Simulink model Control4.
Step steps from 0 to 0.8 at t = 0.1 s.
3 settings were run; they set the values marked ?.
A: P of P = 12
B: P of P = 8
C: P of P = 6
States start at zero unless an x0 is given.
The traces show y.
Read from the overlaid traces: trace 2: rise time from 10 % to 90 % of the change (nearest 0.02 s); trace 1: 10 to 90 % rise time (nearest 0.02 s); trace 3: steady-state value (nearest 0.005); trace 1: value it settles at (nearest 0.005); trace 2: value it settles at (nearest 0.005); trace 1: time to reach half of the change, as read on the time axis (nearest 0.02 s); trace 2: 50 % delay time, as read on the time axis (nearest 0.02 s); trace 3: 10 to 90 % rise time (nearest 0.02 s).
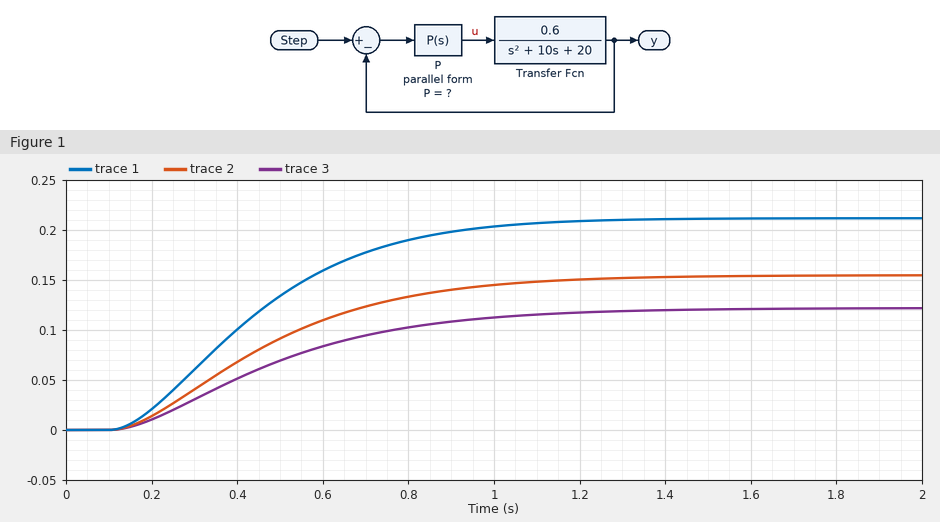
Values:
0.68 s
0.60 s
0.120
0.210
0.155
0.42 s
0.44 s
0.72 s
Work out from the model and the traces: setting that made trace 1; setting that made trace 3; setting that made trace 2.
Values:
A
C
B
